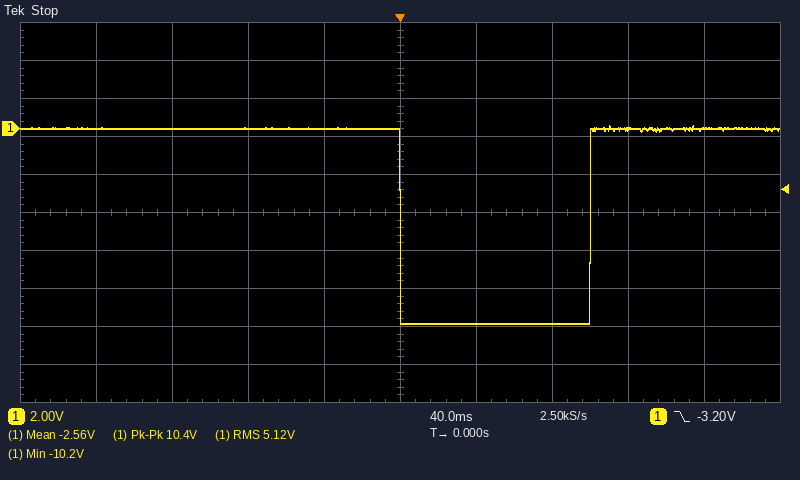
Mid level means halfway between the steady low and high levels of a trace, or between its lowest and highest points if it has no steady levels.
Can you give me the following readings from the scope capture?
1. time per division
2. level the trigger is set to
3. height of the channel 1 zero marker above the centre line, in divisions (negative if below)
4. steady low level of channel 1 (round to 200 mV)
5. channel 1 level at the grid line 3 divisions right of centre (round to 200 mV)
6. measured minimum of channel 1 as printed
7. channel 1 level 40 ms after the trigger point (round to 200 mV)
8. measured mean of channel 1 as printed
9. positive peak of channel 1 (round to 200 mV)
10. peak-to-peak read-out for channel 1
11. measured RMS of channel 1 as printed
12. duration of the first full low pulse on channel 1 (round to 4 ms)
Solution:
40 ms
-3.20 V
+2.2 div
-10.2 V
0.0 V
-10.2 V
-10.2 V
-2.56 V
200 mV
10.4 V
5.12 V
100 ms
